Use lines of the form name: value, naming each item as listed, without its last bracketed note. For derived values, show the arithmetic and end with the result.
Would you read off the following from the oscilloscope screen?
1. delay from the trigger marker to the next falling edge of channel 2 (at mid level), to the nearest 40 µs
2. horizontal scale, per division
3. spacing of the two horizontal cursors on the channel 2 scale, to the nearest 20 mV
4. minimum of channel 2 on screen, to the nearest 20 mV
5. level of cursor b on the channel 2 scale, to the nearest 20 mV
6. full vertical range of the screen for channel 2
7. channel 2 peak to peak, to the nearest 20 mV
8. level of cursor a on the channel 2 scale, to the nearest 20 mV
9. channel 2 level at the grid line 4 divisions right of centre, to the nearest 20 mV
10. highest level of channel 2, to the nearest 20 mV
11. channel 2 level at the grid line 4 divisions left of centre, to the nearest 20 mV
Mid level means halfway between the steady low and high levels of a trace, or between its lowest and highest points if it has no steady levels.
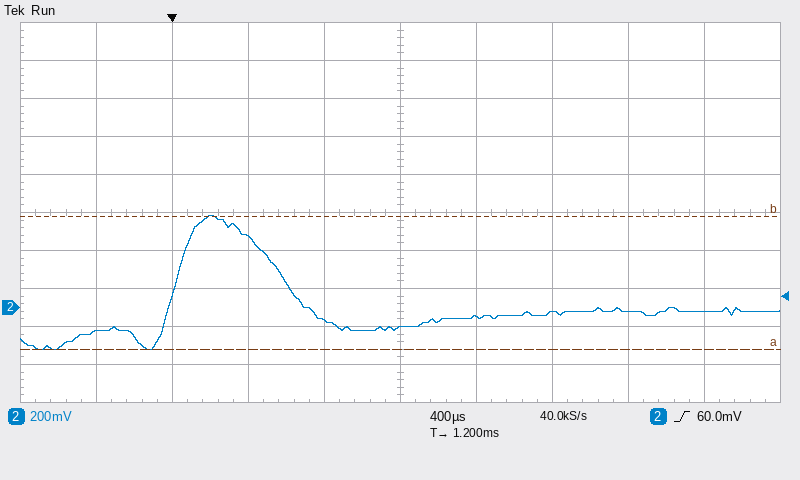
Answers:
delay from the trigger marker to the next falling edge of channel 2 (at mid level), to the nearest 40 µs: 600 µs
horizontal scale, per division: 400 µs
spacing of the two horizontal cursors on the channel 2 scale, to the nearest 20 mV: 700 mV
minimum of channel 2 on screen, to the nearest 20 mV: -220 mV
level of cursor b on the channel 2 scale, to the nearest 20 mV: 480 mV
full vertical range of the screen for channel 2: 2 V
channel 2 peak to peak, to the nearest 20 mV: 480 mV − (-220 mV) = 700 mV
level of cursor a on the channel 2 scale, to the nearest 20 mV: -220 mV
channel 2 level at the grid line 4 divisions right of centre, to the nearest 20 mV: -20 mV
highest level of channel 2, to the nearest 20 mV: 480 mV
channel 2 level at the grid line 4 divisions left of centre, to the nearest 20 mV: -120 mV
